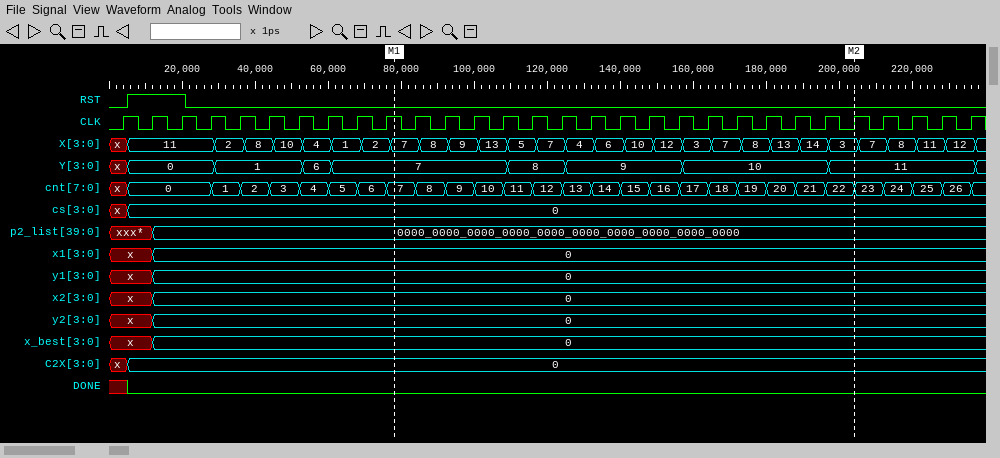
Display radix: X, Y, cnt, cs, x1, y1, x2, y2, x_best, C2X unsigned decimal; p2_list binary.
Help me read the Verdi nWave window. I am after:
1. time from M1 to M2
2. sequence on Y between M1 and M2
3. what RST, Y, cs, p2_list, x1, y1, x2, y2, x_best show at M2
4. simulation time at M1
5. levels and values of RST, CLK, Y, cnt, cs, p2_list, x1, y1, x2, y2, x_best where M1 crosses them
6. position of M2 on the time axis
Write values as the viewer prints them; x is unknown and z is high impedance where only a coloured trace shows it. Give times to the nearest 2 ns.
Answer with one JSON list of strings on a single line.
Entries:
["126 ns", "7, 8, 9, 10, 11", "RST=0, Y=11, cs=0, p2_list=0000_0000_0000_0000_0000_0000_0000_0000_0000_0000, x1=0, y1=0, x2=0, y2=0, x_best=0", "78 ns", "RST=0, CLK=1, Y=7, cnt=7, cs=0, p2_list=0000_0000_0000_0000_0000_0000_0000_0000_0000_0000, x1=0, y1=0, x2=0, y2=0, x_best=0", "204 ns"]
